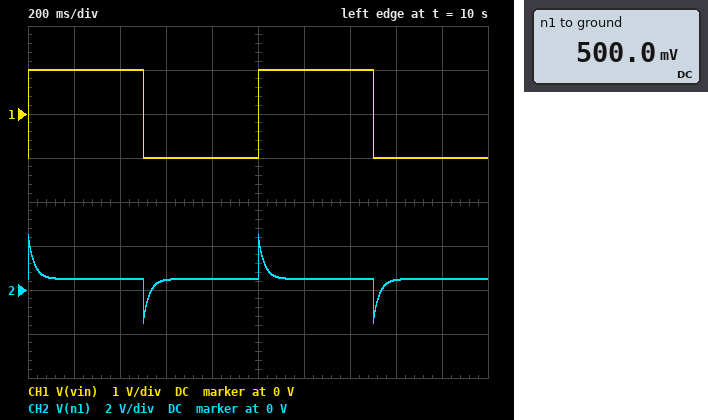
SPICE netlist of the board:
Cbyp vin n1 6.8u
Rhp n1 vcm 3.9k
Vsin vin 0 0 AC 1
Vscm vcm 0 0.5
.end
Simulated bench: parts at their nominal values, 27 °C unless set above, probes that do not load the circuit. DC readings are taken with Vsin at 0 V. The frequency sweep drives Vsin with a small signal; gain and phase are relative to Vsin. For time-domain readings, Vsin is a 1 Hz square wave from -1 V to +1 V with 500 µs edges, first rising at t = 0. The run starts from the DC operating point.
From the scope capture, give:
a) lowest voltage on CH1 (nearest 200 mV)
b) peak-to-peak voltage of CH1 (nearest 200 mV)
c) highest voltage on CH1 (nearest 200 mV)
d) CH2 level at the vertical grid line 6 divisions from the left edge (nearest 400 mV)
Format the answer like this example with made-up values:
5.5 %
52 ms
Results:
-1.0 V
2.0 V
1.0 V
400 mV
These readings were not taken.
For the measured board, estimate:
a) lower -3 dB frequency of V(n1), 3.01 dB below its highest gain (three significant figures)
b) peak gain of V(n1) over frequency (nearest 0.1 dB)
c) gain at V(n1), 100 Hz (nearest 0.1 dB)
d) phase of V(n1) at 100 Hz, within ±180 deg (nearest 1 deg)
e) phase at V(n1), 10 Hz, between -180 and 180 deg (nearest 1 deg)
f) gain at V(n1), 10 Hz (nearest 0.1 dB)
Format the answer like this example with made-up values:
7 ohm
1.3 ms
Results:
6.00 Hz
0 dB
0 dB
3 deg
31 deg
-1.3 dB
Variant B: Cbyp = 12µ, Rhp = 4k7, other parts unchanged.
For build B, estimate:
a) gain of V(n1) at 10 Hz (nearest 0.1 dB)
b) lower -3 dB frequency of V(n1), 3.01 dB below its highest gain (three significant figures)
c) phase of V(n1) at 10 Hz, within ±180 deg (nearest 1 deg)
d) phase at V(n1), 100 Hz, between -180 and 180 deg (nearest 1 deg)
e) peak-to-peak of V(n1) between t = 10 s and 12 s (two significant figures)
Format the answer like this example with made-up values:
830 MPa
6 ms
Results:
-0.3 dB
2.82 Hz
16 deg
2 deg
4.0 V
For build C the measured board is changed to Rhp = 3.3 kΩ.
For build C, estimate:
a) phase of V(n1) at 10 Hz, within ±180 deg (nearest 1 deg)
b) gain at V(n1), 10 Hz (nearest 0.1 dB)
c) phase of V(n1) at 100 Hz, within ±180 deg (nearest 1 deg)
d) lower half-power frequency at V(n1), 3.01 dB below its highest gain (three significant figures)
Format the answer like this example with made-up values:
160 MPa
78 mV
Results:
35 deg
-1.8 dB
4 deg
7.09 Hz
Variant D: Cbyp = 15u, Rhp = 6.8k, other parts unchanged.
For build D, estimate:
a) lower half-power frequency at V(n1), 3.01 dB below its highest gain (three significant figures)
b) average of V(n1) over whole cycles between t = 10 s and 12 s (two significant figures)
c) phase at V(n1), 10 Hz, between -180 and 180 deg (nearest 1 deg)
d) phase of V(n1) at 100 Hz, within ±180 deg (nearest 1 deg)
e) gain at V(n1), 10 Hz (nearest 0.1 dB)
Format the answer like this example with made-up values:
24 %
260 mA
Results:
1.56 Hz
500 mV
9 deg
1 deg
-0.1 dB
